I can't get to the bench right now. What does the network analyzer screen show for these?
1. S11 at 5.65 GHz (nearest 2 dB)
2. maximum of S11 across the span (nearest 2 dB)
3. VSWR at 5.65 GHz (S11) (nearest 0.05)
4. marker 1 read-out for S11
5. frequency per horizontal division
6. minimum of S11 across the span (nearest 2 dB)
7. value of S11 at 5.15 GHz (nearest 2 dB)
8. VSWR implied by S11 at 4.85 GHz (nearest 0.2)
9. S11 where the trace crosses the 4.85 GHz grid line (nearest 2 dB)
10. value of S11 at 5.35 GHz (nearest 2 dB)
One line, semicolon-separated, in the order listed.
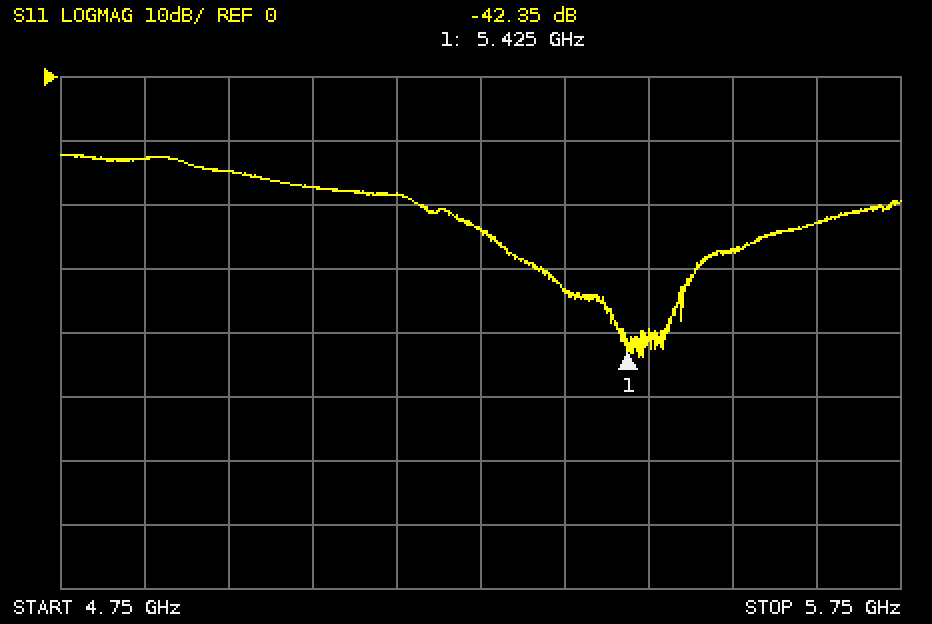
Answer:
-22 dB; -12 dB; 1.15; -42.35 dB; 100 MHz; -44 dB; -18 dB; 1.6; -12 dB; -34 dB
